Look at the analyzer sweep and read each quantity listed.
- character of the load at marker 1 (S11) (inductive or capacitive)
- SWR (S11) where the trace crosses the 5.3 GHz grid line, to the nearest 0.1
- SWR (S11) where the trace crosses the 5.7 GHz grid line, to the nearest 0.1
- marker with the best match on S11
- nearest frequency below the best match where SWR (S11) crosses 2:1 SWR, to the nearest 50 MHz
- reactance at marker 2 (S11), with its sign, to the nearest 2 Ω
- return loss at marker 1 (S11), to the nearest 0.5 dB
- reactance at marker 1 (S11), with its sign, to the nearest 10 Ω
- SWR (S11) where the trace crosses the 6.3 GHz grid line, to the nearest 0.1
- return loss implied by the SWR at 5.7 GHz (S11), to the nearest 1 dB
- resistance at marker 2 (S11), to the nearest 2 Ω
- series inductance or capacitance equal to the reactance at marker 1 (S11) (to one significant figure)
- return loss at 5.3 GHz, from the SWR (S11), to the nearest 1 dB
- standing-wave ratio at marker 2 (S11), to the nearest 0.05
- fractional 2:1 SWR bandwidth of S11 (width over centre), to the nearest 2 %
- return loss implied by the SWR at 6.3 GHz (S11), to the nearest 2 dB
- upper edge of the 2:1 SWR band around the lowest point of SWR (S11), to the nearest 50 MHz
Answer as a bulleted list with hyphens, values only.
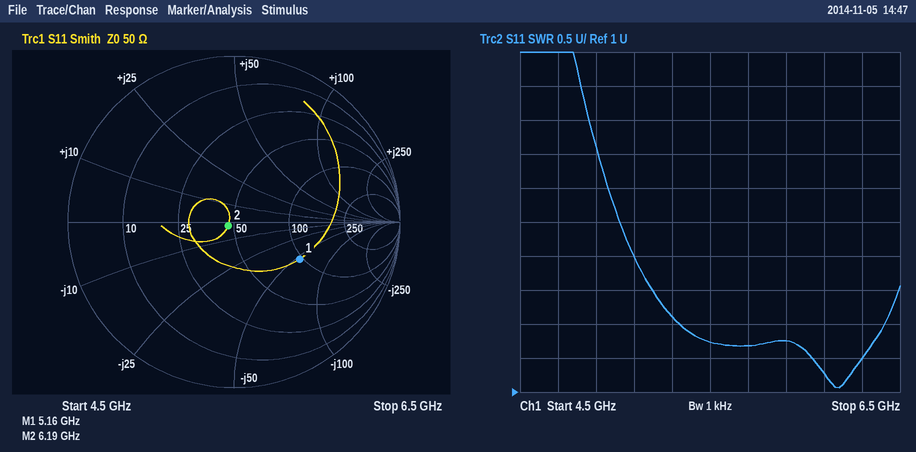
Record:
- capacitive
- 2.1
- 1.7
- marker 2
- 5.35 GHz
- -2 Ω
- 7.0 dB
- -50 Ω
- 1.5
- 12 dB
- 46 Ω
- 600 fF
- 9 dB
- 1.10
- 18 %
- 14 dB
- 6.40 GHz
